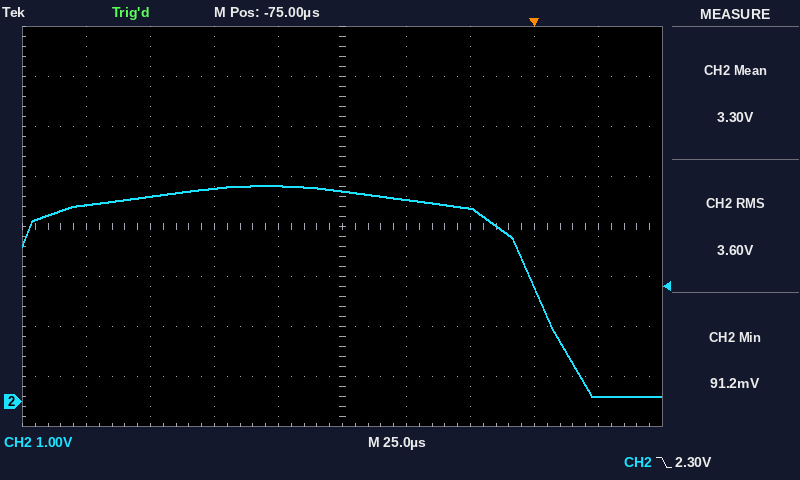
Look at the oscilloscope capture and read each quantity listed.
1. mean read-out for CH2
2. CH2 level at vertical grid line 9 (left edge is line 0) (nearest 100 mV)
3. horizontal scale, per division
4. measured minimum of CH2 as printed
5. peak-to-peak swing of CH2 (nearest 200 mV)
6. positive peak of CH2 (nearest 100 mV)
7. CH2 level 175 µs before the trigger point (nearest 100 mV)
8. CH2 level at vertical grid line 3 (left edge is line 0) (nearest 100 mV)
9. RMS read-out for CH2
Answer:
3.30 V
100 mV
25 µs
91.2 mV
4.2 V
4.3 V
3.9 V
4.3 V
3.60 V
